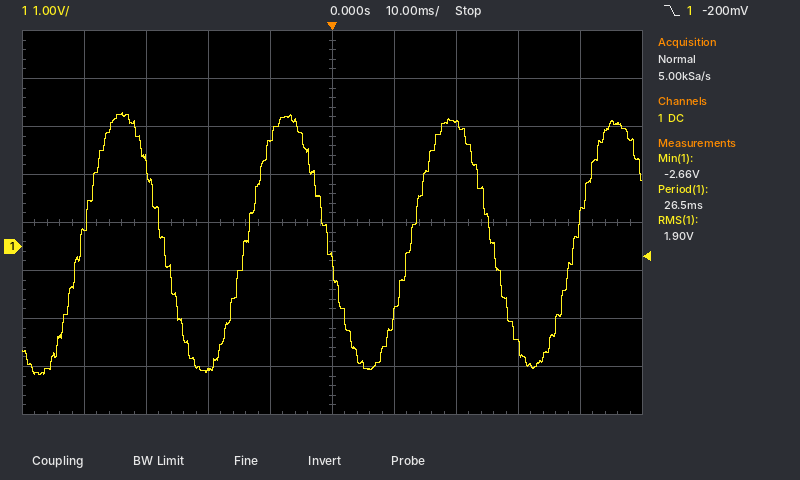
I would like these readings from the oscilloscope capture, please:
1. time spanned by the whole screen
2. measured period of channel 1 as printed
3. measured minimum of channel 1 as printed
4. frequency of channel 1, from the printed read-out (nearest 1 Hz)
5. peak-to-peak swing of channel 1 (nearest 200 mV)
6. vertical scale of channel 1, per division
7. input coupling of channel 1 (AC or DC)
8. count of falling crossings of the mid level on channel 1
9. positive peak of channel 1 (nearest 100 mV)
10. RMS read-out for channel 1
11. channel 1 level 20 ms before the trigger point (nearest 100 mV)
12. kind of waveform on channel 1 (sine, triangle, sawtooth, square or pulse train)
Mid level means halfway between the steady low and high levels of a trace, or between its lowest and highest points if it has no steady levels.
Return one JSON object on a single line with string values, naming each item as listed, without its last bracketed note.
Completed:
{"time spanned by the whole screen": "100 ms", "measured period of channel 1 as printed": "26.5 ms", "measured minimum of channel 1 as printed": "-2.66 V", "frequency of channel 1, from the printed read-out": "38 Hz", "peak-to-peak swing of channel 1": "5.4 V", "vertical scale of channel 1, per division": "1 V", "input coupling of channel 1": "DC", "count of falling crossings of the mid level on channel 1": "3", "positive peak of channel 1": "2.8 V", "RMS read-out for channel 1": "1.90 V", "channel 1 level 20 ms before the trigger point": "-2.6 V", "kind of waveform on channel 1": "sine"}
